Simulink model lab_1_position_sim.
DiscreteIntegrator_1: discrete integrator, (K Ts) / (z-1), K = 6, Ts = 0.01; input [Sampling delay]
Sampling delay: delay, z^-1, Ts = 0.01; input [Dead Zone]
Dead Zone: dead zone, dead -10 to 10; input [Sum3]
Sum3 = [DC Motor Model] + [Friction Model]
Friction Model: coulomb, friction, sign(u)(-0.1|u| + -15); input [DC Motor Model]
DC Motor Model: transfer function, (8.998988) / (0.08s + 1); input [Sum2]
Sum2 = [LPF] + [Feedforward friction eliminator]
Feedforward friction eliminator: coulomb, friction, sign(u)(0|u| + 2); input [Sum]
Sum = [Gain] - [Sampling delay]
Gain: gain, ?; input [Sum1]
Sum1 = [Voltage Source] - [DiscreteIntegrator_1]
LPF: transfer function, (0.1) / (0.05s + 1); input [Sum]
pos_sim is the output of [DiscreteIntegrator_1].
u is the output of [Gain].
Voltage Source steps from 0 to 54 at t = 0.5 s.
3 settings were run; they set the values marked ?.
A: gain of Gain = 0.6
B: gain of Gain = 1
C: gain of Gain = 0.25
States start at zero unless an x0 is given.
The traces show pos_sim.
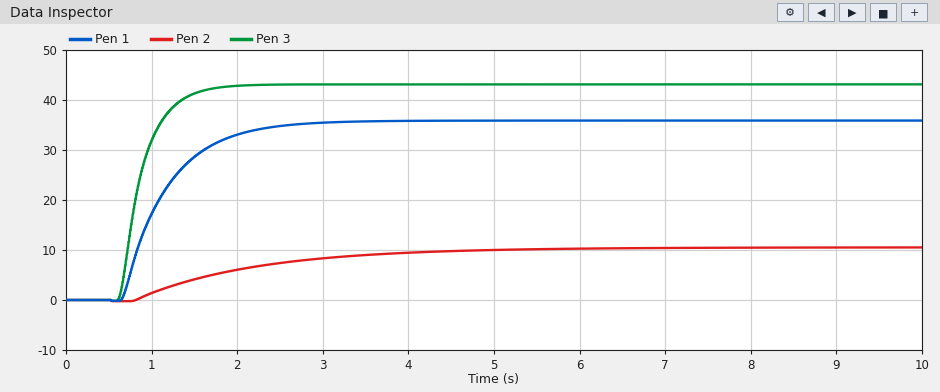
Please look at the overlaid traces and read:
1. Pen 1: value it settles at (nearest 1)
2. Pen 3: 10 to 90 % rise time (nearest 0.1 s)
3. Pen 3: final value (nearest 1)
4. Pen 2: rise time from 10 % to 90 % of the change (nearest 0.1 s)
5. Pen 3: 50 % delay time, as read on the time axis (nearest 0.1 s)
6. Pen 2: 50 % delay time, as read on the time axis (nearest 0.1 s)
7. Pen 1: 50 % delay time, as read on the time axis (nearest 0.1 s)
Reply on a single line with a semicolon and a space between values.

36; 0.6 s; 43; 3.1 s; 0.8 s; 1.8 s; 1.0 s
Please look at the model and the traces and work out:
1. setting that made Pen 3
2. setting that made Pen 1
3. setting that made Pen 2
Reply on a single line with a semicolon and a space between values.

B; A; C
